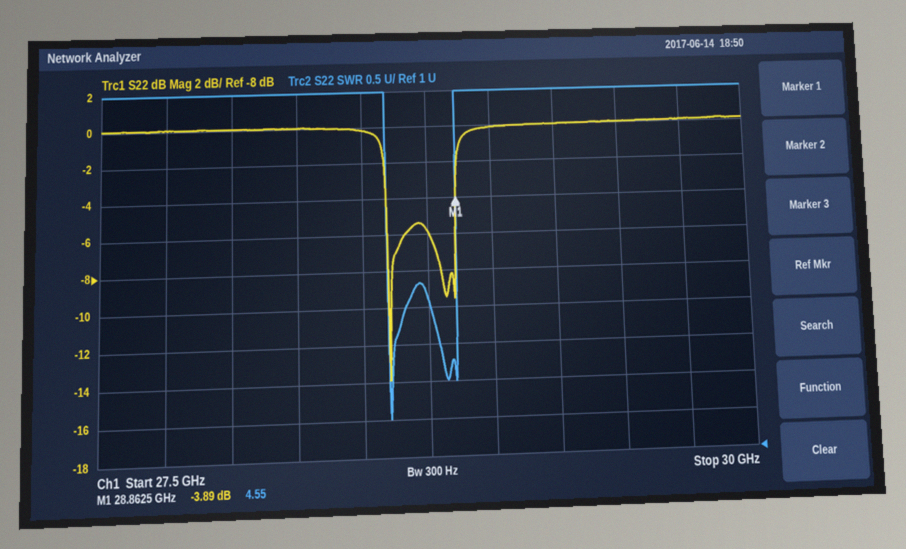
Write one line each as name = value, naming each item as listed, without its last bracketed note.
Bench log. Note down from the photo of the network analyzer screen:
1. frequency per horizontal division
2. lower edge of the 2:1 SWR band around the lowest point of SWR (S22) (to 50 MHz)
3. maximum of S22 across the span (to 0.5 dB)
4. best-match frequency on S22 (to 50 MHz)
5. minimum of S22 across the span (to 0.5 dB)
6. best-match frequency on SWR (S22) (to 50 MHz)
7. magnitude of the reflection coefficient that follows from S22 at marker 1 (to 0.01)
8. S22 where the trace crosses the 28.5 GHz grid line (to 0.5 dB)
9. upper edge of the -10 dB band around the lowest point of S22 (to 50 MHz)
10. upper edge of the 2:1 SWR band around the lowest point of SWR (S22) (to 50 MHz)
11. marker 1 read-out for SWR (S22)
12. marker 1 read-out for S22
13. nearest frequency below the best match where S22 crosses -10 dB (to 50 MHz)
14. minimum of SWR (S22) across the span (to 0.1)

frequency per horizontal division = 250 MHz
lower edge of the 2:1 SWR band around the lowest point of SWR (S22) = 28.60 GHz
maximum of S22 across the span = 0.0 dB
best-match frequency on S22 = 28.60 GHz
minimum of S22 across the span = -14.0 dB
best-match frequency on SWR (S22) = 28.60 GHz
magnitude of the reflection coefficient that follows from S22 at marker 1 = 0.64
S22 where the trace crosses the 28.5 GHz grid line = 0.0 dB
upper edge of the -10 dB band around the lowest point of S22 = 28.60 GHz
upper edge of the 2:1 SWR band around the lowest point of SWR (S22) = 28.60 GHz
marker 1 read-out for SWR = 4.55
marker 1 read-out for S22 = -3.89 dB
nearest frequency below the best match where S22 crosses -10 dB = 28.60 GHz
minimum of SWR (S22) across the span = 1.5
